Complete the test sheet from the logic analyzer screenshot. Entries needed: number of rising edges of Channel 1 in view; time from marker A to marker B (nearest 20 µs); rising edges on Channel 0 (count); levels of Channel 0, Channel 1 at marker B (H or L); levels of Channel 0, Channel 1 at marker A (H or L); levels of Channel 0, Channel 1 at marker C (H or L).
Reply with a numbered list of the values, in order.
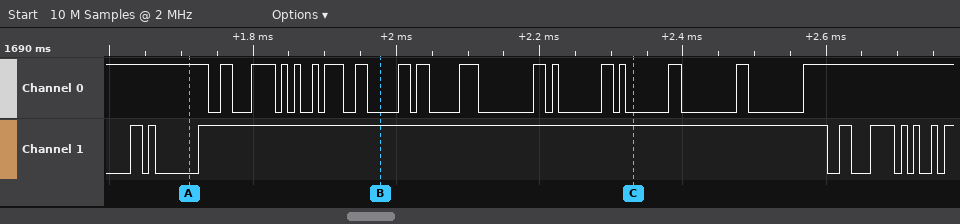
1. 9
2. 260 µs
3. 17
4. Channel 0=L, Channel 1=H
5. Channel 0=H, Channel 1=L
6. Channel 0=L, Channel 1=H
